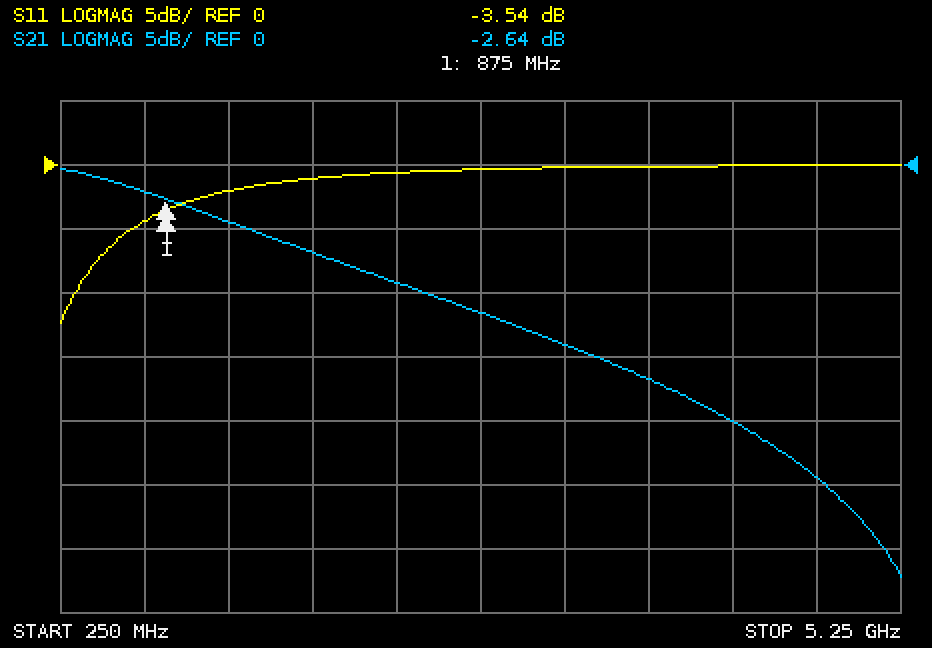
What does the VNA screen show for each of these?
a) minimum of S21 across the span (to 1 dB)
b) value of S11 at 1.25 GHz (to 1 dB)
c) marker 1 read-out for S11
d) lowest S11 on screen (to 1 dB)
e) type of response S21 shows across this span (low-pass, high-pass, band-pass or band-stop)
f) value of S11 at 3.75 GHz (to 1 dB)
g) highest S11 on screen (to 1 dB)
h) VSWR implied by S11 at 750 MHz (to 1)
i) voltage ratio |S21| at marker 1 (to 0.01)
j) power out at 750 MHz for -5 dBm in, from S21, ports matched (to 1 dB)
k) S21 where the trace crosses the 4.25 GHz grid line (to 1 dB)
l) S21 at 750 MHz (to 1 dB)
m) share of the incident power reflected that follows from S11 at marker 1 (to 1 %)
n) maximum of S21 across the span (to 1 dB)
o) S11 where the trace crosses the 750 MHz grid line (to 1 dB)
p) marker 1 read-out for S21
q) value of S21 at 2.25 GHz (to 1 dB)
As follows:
-32 dB
-2 dB
-3.54 dB
-12 dB
low-pass
0 dB
0 dB
4
0.74
-7 dBm
-20 dB
-2 dB
44 %
0 dB
-4 dB
-2.64 dB
-9 dB
